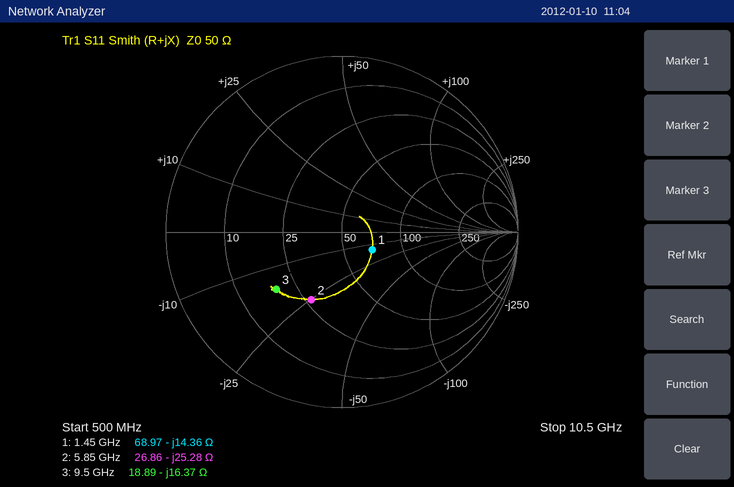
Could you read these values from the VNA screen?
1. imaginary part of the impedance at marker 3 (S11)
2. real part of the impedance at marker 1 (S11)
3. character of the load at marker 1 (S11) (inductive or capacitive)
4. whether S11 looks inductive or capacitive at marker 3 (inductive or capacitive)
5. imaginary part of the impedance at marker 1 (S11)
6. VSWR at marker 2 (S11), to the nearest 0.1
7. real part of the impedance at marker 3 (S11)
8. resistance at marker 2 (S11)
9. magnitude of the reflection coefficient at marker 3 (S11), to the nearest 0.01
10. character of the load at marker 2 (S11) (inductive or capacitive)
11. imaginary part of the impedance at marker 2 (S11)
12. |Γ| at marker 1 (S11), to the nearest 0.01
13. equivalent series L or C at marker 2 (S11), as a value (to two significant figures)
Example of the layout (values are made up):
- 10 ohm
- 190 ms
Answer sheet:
- -16.37 Ω
- 68.97 Ω
- capacitive
- capacitive
- -14.36 Ω
- 2.5
- 18.89 Ω
- 26.86 Ω
- 0.50
- capacitive
- -25.28 Ω
- 0.20
- 1.1 pF
